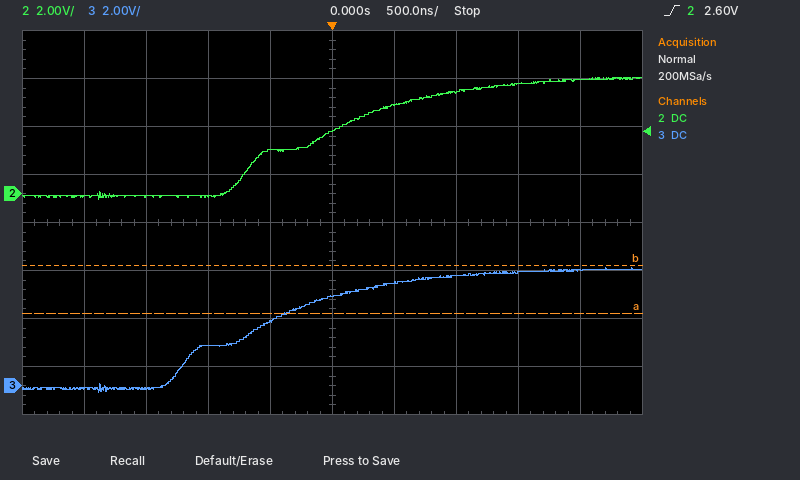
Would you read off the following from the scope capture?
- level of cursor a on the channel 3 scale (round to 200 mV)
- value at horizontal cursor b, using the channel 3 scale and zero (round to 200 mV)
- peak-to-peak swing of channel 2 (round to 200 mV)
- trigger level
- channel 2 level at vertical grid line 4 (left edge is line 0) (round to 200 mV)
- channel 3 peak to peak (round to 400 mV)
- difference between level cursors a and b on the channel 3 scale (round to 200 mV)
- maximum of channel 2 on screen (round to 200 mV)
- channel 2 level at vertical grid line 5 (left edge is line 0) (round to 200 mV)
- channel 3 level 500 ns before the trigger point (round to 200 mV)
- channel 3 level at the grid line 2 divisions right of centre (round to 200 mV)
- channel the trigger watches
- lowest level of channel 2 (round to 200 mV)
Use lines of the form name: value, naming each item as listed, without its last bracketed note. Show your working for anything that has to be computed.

level of cursor a on the channel 3 scale: 3.0 V
value at horizontal cursor b, using the channel 3 scale and zero: 5.0 V
peak-to-peak swing of channel 2: 4.8 V − (-200 mV) = 5.0 V
trigger level: 2.60 V
channel 2 level at vertical grid line 4 (left edge is line 0): 1.8 V
channel 3 peak to peak: 5.2 V
difference between level cursors a and b on the channel 3 scale: 2.0 V
maximum of channel 2 on screen: 4.8 V
channel 2 level at vertical grid line 5 (left edge is line 0): 2.6 V
channel 3 level 500 ns before the trigger point: 2.6 V
channel 3 level at the grid line 2 divisions right of centre: 4.6 V
channel the trigger watches: channel 2
lowest level of channel 2: -200 mV
